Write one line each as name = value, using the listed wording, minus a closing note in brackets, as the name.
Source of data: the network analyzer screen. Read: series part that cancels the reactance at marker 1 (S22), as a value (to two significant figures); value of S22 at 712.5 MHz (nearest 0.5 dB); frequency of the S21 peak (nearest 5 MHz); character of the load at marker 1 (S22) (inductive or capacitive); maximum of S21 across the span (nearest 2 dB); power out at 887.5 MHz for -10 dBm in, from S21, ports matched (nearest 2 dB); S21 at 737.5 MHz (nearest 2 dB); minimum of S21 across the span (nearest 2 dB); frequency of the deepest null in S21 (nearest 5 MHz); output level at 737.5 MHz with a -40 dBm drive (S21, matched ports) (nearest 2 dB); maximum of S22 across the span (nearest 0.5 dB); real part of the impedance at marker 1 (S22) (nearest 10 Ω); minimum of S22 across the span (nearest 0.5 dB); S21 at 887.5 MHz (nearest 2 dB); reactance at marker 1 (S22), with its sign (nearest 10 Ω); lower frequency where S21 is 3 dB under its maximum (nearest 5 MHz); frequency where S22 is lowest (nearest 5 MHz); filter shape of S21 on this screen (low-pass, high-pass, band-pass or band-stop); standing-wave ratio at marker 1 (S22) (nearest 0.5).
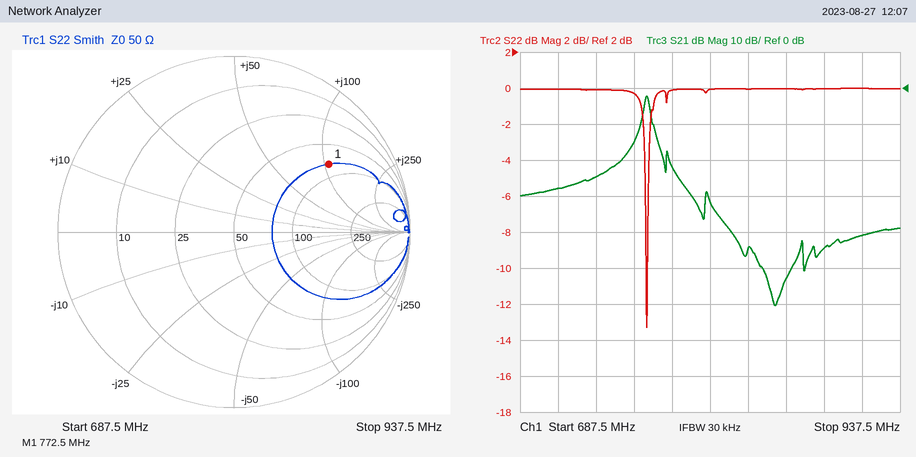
series part that cancels the reactance at marker 1 (S22), as a value = 1.9 pF
value of S22 at 712.5 MHz = 0.0 dB
frequency of the S21 peak = 770 MHz
character of the load at marker 1 (S22) = inductive
maximum of S21 across the span = -2 dB
power out at 887.5 MHz for -10 dBm in, from S21, ports matched = -54 dBm
S21 at 737.5 MHz = -24 dB
minimum of S21 across the span = -60 dB
frequency of the deepest null in S21 = 855 MHz
output level at 737.5 MHz with a -40 dBm drive (S21, matched ports) = -64 dBm
maximum of S22 across the span = 0.0 dB
real part of the impedance at marker 1 (S22) = 80 Ω
minimum of S22 across the span = -13.5 dB
S21 at 887.5 MHz = -44 dB
reactance at marker 1 (S22), with its sign = +110 Ω
lower frequency where S21 is 3 dB under its maximum = 770 MHz
frequency where S22 is lowest = 770 MHz
filter shape of S21 on this screen = band-pass
standing-wave ratio at marker 1 (S22) = 5.0
